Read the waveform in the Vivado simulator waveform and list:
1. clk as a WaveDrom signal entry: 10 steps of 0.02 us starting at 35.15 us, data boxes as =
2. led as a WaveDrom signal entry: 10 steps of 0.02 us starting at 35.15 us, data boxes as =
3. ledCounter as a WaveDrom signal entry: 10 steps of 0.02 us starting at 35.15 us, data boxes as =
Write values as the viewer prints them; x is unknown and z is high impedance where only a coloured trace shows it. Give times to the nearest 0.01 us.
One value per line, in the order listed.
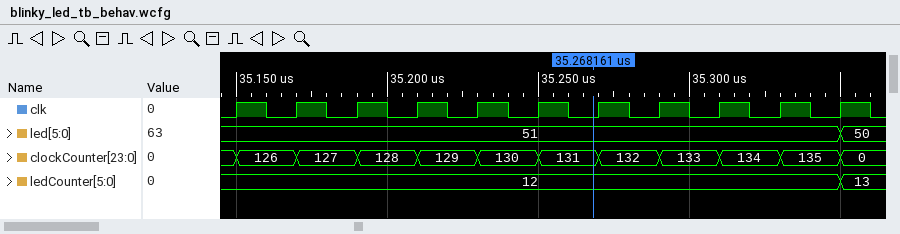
{name: 'clk', wave: 'p.........'}
{name: 'led', wave: '=.........', data: '51'}
{name: 'ledCounter', wave: '=.........', data: '12'}
